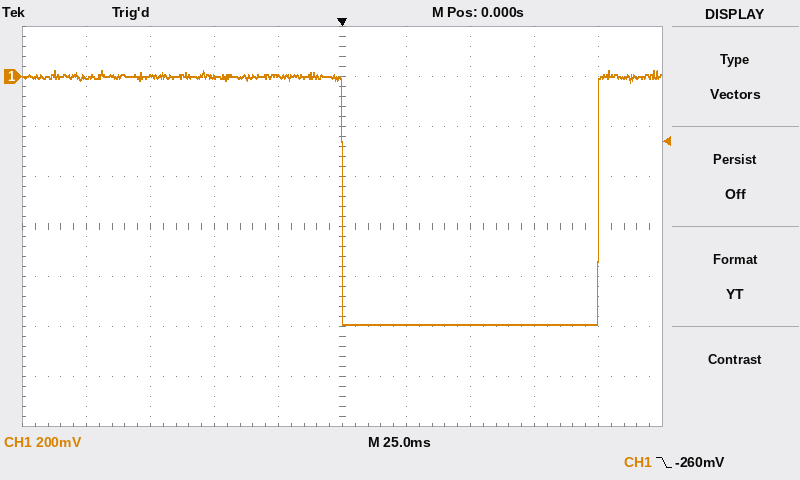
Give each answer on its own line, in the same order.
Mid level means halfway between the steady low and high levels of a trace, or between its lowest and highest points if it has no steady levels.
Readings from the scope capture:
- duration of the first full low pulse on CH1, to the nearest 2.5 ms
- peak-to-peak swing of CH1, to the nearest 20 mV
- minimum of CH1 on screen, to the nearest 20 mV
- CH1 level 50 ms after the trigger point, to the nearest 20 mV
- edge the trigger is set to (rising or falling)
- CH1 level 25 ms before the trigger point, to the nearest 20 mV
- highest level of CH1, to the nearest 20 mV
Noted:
100.0 ms
1.02 V
-1.00 V
-1.00 V
falling
0 mV
20 mV
